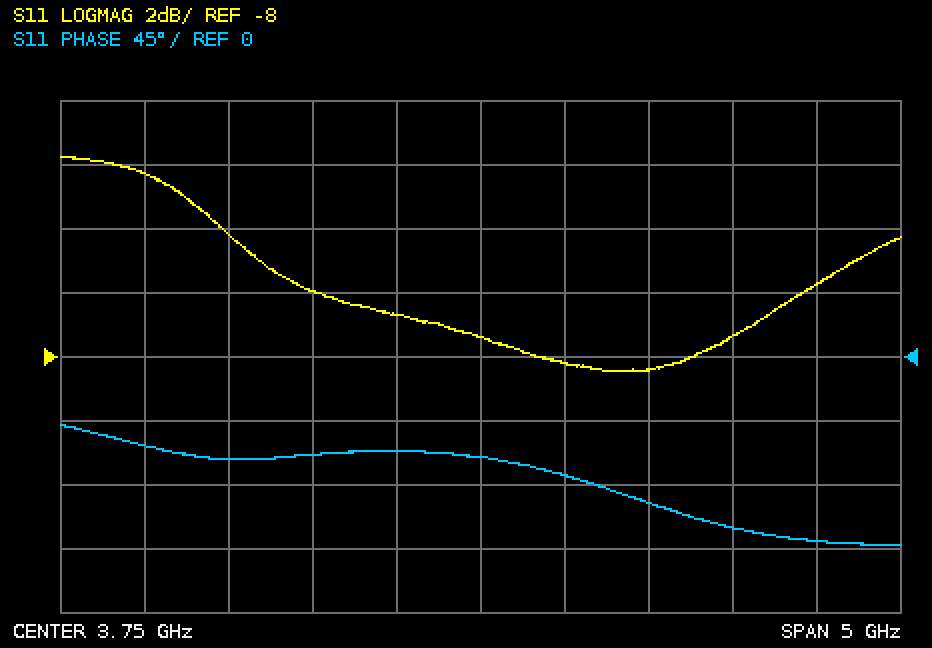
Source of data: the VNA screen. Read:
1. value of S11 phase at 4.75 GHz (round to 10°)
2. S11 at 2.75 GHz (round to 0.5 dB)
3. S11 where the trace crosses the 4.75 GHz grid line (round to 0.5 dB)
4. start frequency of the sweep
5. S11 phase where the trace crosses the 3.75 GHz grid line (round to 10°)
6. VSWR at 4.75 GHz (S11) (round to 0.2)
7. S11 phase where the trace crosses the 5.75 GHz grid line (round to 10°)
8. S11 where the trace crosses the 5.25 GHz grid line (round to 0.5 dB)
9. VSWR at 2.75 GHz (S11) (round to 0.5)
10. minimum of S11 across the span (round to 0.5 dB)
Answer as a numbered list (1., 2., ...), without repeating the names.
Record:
1. -100°
2. -6.0 dB
3. -8.5 dB
4. 1.25 GHz
5. -70°
6. 2.2
7. -130°
8. -7.5 dB
9. 3.0
10. -8.5 dB
